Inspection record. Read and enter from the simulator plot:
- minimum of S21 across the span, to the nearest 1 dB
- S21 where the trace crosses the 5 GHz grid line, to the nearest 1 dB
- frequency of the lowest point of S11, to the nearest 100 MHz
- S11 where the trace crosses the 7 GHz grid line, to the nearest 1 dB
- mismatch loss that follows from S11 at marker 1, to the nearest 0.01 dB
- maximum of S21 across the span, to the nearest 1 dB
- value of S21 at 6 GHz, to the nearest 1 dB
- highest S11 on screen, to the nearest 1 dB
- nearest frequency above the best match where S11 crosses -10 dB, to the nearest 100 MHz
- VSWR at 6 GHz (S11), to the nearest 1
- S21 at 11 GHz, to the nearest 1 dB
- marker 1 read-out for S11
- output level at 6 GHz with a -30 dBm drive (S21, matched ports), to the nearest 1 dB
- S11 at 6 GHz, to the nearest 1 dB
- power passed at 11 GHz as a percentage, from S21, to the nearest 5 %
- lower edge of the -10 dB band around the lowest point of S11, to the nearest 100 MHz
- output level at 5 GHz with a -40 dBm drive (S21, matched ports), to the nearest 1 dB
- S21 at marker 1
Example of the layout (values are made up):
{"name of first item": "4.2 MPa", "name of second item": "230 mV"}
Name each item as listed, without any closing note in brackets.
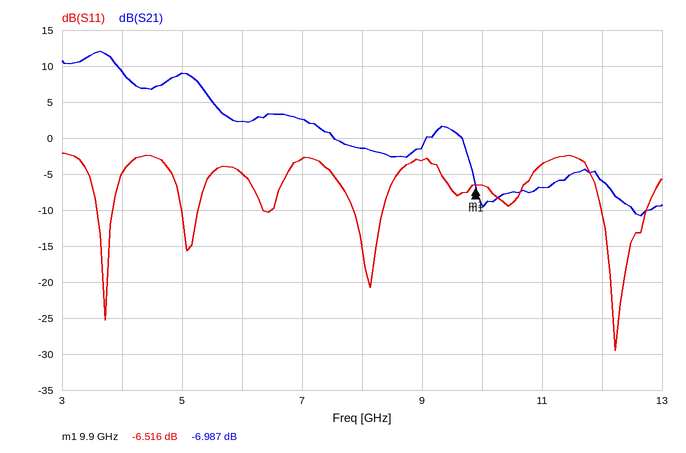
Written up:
{"minimum of S21 across the span, to the nearest 1 dB": "-11 dB", "S21 where the trace crosses the 5 GHz grid line, to the nearest 1 dB": "9 dB", "frequency of the lowest point of S11, to the nearest 100 MHz": "12.2 GHz", "S11 where the trace crosses the 7 GHz grid line, to the nearest 1 dB": "-3 dB", "mismatch loss that follows from S11 at marker 1, to the nearest 0.01 dB": "1.10 dB", "maximum of S21 across the span, to the nearest 1 dB": "12 dB", "value of S21 at 6 GHz, to the nearest 1 dB": "2 dB", "highest S11 on screen, to the nearest 1 dB": "-2 dB", "nearest frequency above the best match where S11 crosses -10 dB, to the nearest 100 MHz": "12.7 GHz", "VSWR at 6 GHz (S11), to the nearest 1": "4", "S21 at 11 GHz, to the nearest 1 dB": "-7 dB", "marker 1 read-out for S11": "-6.516 dB", "output level at 6 GHz with a -30 dBm drive (S21, matched ports), to the nearest 1 dB": "-28 dBm", "S11 at 6 GHz, to the nearest 1 dB": "-5 dB", "power passed at 11 GHz as a percentage, from S21, to the nearest 5 %": "20 %", "lower edge of the -10 dB band around the lowest point of S11, to the nearest 100 MHz": "12.0 GHz", "output level at 5 GHz with a -40 dBm drive (S21, matched ports), to the nearest 1 dB": "-31 dBm", "S21 at marker 1": "-6.987 dB"}
